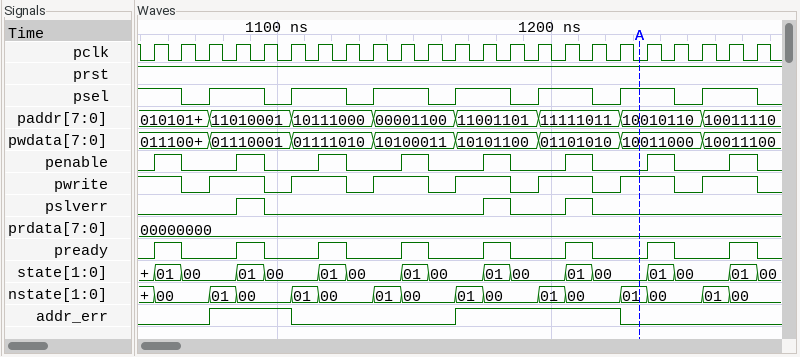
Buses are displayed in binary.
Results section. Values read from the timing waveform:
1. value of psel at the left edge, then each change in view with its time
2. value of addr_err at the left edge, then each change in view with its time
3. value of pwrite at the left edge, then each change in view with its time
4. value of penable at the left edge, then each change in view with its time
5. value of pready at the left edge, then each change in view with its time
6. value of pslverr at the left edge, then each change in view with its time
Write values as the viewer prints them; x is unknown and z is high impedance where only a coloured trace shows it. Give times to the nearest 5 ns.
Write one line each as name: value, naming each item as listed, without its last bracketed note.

value of psel at the left edge, then each change in view with its time: 1, 0 at 1065 ns, 1 at 1075 ns, 0 at 1095 ns, 1 at 1105 ns, 0 at 1125 ns, 1 at 1135 ns, 0 at 1155 ns, 1 at 1165 ns, 0 at 1185 ns, 1 at 1195 ns, 0 at 1215 ns, 1 at 1225 ns, 0 at 1245 ns, 1 at 1255 ns, 0 at 1275 ns
value of addr_err at the left edge, then each change in view with its time: 0, 1 at 1075 ns, 0 at 1105 ns, 1 at 1165 ns, 0 at 1225 ns
value of pwrite at the left edge, then each change in view with its time: 1, 0 at 1065 ns, 1 at 1075 ns, 0 at 1095 ns, 1 at 1105 ns, 0 at 1125 ns, 1 at 1135 ns, 0 at 1155 ns, 1 at 1165 ns, 0 at 1185 ns, 1 at 1195 ns, 0 at 1215 ns, 1 at 1225 ns, 0 at 1245 ns, 1 at 1255 ns, 0 at 1275 ns
value of penable at the left edge, then each change in view with its time: 0, 1 at 1055 ns, 0 at 1065 ns, 1 at 1085 ns, 0 at 1095 ns, 1 at 1115 ns, 0 at 1125 ns, 1 at 1145 ns, 0 at 1155 ns, 1 at 1175 ns, 0 at 1185 ns, 1 at 1205 ns, 0 at 1215 ns, 1 at 1235 ns, 0 at 1245 ns, 1 at 1265 ns, 0 at 1275 ns
value of pready at the left edge, then each change in view with its time: 0, 1 at 1055 ns, 0 at 1065 ns, 1 at 1085 ns, 0 at 1095 ns, 1 at 1115 ns, 0 at 1125 ns, 1 at 1145 ns, 0 at 1155 ns, 1 at 1175 ns, 0 at 1185 ns, 1 at 1205 ns, 0 at 1215 ns, 1 at 1235 ns, 0 at 1245 ns, 1 at 1265 ns, 0 at 1275 ns
value of pslverr at the left edge, then each change in view with its time: 0, 1 at 1085 ns, 0 at 1095 ns, 1 at 1175 ns, 0 at 1185 ns, 1 at 1205 ns, 0 at 1215 ns
